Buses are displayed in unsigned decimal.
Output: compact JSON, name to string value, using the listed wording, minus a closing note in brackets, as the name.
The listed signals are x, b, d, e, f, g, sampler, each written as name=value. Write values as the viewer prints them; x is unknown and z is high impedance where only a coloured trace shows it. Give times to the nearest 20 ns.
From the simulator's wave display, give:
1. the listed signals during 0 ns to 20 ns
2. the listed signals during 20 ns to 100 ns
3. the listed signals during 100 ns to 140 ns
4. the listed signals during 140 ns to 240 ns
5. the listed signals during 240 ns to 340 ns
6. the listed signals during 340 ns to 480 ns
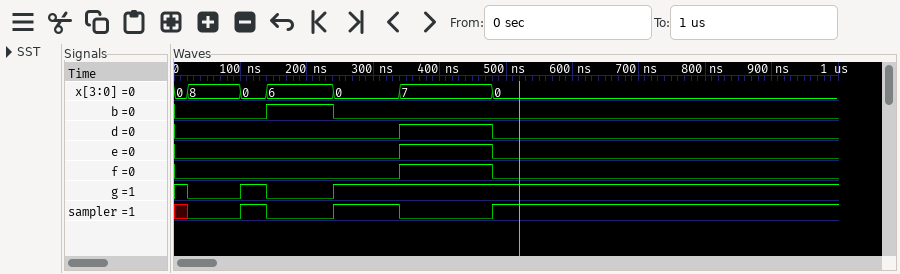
{"the listed signals during 0 ns to 20 ns": "x=0, b=0, d=0, e=0, f=0, g=1, sampler=x", "the listed signals during 20 ns to 100 ns": "x=8, b=0, d=0, e=0, f=0, g=0, sampler=0", "the listed signals during 100 ns to 140 ns": "x=0, b=0, d=0, e=0, f=0, g=1, sampler=1", "the listed signals during 140 ns to 240 ns": "x=6, b=1, d=0, e=0, f=0, g=0, sampler=0", "the listed signals during 240 ns to 340 ns": "x=0, b=0, d=0, e=0, f=0, g=1, sampler=1", "the listed signals during 340 ns to 480 ns": "x=7, b=0, d=1, e=1, f=1, g=1, sampler=0"}
